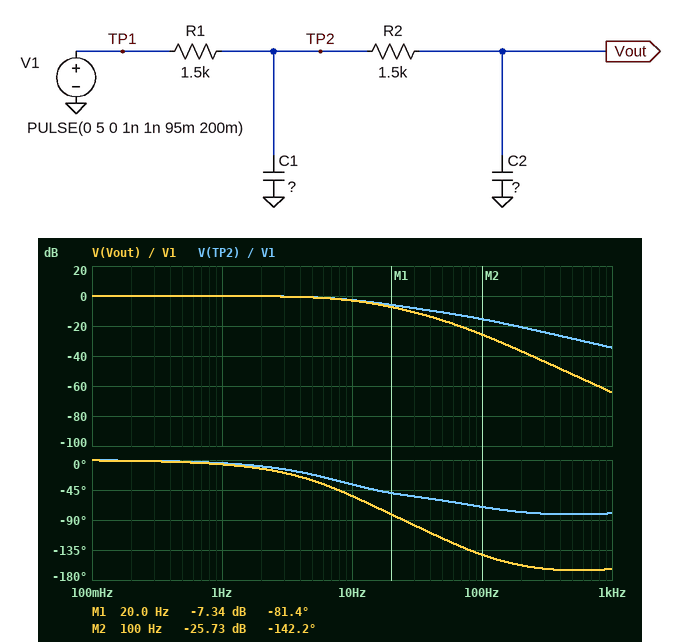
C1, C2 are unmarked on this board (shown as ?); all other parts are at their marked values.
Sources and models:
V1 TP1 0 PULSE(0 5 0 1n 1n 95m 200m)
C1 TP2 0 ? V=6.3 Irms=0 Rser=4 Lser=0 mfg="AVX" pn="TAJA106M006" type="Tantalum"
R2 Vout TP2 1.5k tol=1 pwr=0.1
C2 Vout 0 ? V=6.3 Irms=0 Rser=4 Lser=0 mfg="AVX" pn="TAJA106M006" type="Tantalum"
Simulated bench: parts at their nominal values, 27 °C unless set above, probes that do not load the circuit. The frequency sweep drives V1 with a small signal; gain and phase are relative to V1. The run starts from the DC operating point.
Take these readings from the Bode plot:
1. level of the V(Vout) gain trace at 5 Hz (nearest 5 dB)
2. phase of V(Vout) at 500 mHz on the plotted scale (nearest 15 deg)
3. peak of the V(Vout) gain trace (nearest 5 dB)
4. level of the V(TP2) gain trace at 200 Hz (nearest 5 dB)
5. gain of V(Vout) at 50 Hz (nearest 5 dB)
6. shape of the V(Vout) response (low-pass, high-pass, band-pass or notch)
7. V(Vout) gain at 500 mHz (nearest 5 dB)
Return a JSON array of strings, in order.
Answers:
["0 dB", "0 deg", "0 dB", "-20 dB", "-15 dB", "low-pass", "0 dB"]
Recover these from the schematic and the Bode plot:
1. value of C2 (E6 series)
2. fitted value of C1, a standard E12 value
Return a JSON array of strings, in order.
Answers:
["3.3 µF", "5.6 µF"]
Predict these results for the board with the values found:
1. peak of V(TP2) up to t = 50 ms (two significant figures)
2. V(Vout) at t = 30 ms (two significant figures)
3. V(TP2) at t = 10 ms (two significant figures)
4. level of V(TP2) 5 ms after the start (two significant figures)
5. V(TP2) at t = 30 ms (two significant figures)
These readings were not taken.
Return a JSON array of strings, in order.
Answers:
["4.8 V", "4.1 V", "2.8 V", "1.9 V", "4.4 V"]
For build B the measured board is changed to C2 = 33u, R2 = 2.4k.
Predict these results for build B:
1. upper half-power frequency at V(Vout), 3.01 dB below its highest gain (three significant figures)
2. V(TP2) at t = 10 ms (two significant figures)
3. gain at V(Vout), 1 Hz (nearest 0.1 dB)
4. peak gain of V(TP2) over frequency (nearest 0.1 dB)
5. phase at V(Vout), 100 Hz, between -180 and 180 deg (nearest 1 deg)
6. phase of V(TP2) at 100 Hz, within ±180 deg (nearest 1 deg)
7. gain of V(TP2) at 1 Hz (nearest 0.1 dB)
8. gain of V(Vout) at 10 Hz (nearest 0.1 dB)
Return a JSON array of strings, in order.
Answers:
["1.20 Hz", "2.7 V", "-2.3 dB", "0 dB", "-156 deg", "-72 deg", "-1.3 dB", "-18.9 dB"]
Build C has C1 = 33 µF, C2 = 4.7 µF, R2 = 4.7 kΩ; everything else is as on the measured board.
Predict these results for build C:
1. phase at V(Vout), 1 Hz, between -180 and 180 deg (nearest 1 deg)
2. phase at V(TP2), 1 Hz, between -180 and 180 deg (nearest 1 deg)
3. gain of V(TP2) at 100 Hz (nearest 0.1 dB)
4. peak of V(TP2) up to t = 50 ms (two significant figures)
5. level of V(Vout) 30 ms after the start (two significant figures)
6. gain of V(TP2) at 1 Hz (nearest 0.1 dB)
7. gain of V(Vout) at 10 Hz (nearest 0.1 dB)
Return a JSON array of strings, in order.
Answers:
["-27 deg", "-19 deg", "-29.9 dB", "3.0 V", "1.1 V", "-0.6 dB", "-15.5 dB"]
